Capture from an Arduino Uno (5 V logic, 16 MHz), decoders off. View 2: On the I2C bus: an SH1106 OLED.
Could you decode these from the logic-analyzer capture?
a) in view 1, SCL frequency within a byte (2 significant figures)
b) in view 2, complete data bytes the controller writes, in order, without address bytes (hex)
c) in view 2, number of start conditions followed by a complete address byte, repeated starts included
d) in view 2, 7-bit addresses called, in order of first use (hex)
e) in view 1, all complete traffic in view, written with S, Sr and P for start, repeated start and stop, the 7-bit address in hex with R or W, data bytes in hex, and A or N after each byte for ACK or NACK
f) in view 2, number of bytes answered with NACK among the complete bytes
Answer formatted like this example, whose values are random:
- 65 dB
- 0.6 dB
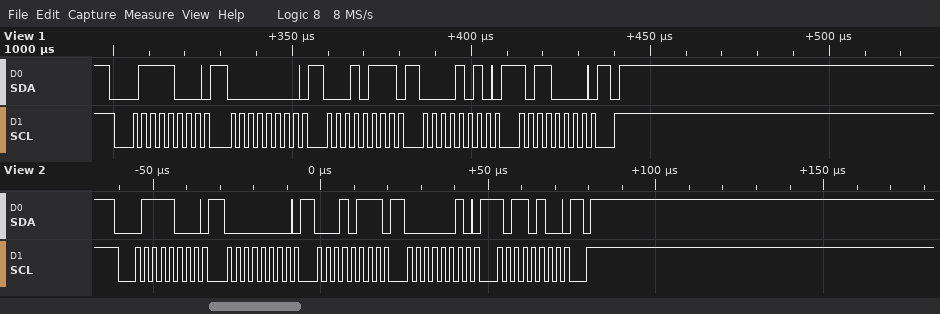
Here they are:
- 400 kHz
- 00 17 02 B4
- 1
- 0x3C
- S 3CW A 00 A 17 A 0A A B0 A P
- 0
